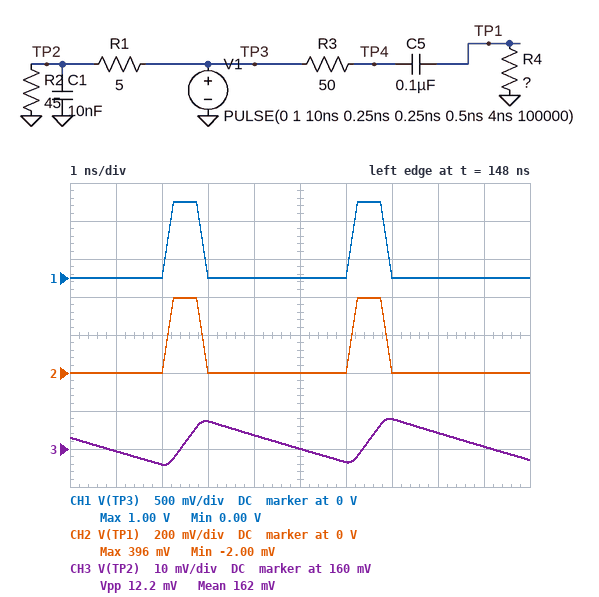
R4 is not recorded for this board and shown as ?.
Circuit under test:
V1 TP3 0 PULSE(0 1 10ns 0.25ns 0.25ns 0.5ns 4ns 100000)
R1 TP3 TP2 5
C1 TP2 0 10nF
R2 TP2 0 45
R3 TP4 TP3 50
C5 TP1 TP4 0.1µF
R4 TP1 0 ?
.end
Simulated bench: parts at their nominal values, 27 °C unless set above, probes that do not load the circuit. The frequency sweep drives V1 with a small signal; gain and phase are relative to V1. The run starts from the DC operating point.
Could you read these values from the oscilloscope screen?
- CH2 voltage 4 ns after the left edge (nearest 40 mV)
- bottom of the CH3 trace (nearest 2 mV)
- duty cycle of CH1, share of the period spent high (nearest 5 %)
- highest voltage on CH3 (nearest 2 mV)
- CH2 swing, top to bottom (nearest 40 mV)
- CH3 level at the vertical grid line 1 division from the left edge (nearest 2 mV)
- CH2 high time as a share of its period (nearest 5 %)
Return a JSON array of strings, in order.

["0 V", "156 mV", "20 %", "168 mV", "400 mV", "160 mV", "20 %"]
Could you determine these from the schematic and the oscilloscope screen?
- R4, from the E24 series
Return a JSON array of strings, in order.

["33 Ω"]
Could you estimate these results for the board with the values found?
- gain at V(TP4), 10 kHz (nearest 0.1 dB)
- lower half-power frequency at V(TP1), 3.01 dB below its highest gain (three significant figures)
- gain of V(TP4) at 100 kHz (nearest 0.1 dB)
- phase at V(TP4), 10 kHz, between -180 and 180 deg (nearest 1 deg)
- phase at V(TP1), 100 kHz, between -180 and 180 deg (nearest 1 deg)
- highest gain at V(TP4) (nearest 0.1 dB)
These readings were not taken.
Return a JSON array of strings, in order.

["-0.9 dB", "19.2 kHz", "-7.3 dB", "-16 deg", "11 deg", "0 dB"]
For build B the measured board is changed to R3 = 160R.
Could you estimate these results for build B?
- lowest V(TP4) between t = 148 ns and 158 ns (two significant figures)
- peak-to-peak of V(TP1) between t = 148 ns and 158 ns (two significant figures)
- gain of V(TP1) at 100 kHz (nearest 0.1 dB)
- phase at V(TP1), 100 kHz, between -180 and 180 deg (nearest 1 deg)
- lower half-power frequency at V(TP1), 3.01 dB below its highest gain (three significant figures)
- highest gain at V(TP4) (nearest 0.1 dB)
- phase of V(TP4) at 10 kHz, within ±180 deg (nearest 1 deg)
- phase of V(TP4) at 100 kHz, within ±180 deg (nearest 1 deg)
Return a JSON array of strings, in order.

["1.1 mV", "170 mV", "-15.4 dB", "5 deg", "8.25 kHz", "0 dB", "-39 deg", "-21 deg"]
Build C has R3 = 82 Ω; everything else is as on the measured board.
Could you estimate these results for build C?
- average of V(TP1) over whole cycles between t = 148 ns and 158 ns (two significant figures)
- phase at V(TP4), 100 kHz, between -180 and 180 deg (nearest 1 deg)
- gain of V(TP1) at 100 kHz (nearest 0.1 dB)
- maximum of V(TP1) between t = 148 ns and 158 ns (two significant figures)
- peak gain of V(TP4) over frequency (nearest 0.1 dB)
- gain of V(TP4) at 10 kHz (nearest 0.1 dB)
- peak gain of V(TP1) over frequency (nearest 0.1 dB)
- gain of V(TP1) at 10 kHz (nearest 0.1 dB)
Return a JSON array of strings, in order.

["53 mV", "-18 deg", "-10.9 dB", "290 mV", "0 dB", "-1.6 dB", "-10.8 dB", "-15.5 dB"]
